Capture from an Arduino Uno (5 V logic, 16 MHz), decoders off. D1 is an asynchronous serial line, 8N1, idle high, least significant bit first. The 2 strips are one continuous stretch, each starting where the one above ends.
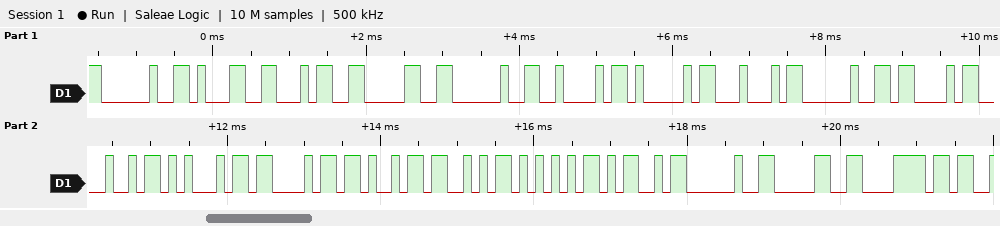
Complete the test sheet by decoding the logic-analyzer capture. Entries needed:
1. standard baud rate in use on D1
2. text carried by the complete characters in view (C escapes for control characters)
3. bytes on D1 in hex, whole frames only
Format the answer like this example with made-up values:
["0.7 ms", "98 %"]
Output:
["9600 baud", "\" 140 BAD CHECKSUM 0x\"", "20 31 34 30 20 42 41 44 20 43 48 45 43 4B 53 55 4D 20 30 78"]
